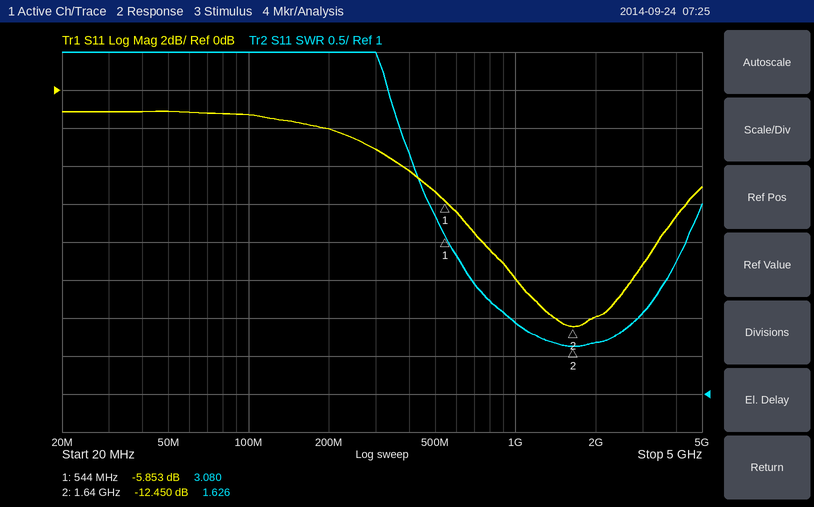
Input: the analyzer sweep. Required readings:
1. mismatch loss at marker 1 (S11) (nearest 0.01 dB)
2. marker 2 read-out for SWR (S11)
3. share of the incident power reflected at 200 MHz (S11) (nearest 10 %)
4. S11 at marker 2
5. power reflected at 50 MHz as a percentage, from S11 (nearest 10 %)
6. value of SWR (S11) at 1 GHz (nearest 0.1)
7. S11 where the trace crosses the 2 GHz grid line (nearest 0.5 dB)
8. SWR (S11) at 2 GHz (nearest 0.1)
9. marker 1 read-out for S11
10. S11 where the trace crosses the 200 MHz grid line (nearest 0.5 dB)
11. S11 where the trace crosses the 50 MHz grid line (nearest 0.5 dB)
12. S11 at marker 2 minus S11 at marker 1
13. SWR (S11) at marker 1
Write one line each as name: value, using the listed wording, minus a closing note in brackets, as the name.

mismatch loss at marker 1 (S11): 1.31 dB
marker 2 read-out for SWR: 1.626
share of the incident power reflected at 200 MHz (S11): 60 %
S11 at marker 2: -12.450 dB
power reflected at 50 MHz as a percentage, from S11: 80 %
value of SWR (S11) at 1 GHz: 1.9
S11 where the trace crosses the 2 GHz grid line: -12.0 dB
SWR (S11) at 2 GHz: 1.7
marker 1 read-out for S11: -5.853 dB
S11 where the trace crosses the 200 MHz grid line: -2.0 dB
S11 where the trace crosses the 50 MHz grid line: -1.0 dB
S11 at marker 2 minus S11 at marker 1: -6.597 dB
SWR (S11) at marker 1: 3.080
